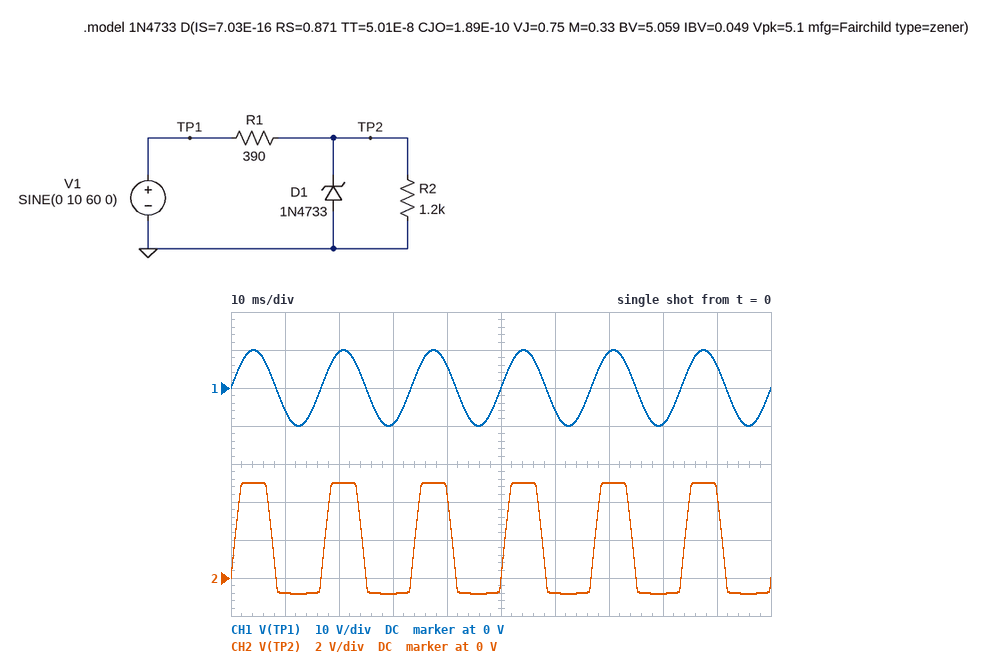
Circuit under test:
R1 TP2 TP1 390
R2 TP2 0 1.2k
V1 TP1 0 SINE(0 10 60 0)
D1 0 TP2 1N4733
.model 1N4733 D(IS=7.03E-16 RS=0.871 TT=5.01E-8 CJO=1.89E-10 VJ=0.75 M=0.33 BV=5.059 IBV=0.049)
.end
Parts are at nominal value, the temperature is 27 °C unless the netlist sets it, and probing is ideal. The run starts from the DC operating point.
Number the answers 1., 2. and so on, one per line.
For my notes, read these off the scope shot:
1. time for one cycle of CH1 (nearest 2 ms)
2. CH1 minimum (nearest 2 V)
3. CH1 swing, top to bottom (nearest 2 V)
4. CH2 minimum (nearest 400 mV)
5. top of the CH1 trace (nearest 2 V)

1. 16 ms
2. -10 V
3. 20 V
4. -800 mV
5. 10 V
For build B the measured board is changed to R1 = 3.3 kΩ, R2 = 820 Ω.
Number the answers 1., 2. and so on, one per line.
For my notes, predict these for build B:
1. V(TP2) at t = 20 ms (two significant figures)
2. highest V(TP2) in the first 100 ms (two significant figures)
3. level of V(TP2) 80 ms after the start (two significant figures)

1. 1.9 V
2. 2.0 V
3. -740 mV
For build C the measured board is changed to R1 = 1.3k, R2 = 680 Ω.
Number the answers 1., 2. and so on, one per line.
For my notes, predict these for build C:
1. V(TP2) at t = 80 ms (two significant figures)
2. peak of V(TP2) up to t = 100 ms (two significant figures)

1. -770 mV
2. 3.4 V
